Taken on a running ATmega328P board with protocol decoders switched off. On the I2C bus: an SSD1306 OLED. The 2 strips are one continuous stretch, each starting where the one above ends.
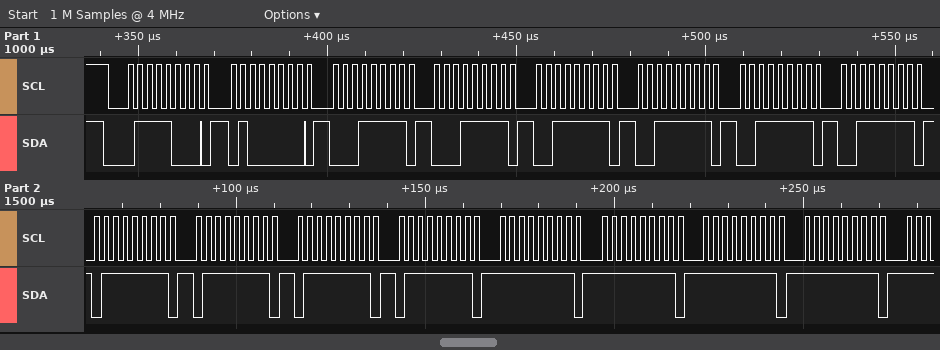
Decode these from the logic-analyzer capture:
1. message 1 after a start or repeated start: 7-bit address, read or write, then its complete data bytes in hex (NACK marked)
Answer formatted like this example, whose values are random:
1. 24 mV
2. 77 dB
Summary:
1. 0x3C write: 40 1F 1F 3F 3F 3F 3F 7F 7F 7F 7F FF FF FF FF
